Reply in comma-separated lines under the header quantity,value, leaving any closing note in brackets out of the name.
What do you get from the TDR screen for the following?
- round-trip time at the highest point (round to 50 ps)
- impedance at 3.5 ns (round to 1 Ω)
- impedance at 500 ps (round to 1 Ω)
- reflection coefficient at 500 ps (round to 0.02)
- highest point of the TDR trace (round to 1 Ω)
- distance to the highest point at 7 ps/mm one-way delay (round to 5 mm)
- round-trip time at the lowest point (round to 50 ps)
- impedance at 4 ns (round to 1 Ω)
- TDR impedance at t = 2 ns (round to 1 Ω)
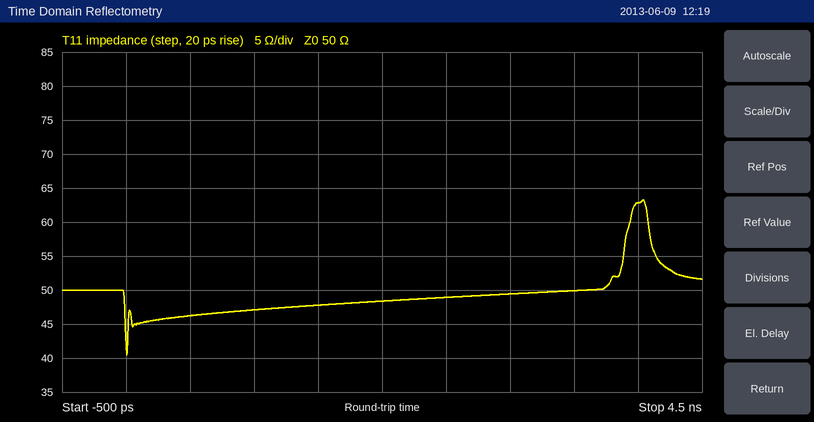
quantity,value
round-trip time at the highest point,4.05 ns
impedance at 3.5 ns,50 Ω
impedance at 500 ps,46 Ω
reflection coefficient at 500 ps,-0.04
highest point of the TDR trace,63 Ω
distance to the highest point at 7 ps/mm one-way delay,290 mm
round-trip time at the lowest point,0 ps
impedance at 4 ns,63 Ω
TDR impedance at t = 2 ns,48 Ω
